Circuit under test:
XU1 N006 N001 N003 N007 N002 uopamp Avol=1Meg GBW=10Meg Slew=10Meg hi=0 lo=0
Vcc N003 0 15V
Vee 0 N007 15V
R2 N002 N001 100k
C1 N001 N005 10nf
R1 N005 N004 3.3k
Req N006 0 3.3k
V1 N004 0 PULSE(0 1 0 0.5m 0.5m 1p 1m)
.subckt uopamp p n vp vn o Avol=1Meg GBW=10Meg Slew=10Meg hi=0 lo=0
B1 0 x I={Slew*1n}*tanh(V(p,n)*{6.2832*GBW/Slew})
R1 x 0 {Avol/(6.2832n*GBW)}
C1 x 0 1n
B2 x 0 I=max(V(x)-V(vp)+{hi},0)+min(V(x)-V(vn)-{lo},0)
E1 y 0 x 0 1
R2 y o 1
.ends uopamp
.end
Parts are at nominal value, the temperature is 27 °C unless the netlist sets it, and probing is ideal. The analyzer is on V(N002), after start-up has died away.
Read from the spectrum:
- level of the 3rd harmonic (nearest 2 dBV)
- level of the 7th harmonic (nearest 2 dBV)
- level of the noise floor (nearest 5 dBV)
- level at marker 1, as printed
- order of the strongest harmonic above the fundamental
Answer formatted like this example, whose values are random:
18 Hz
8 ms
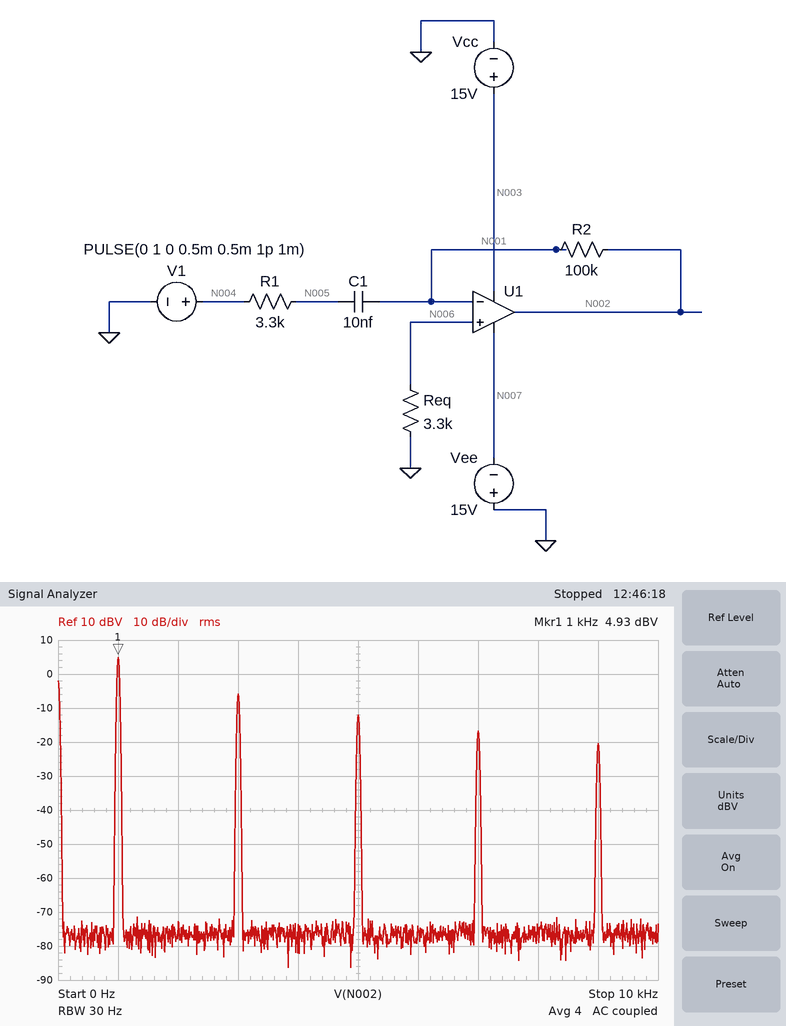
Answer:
-6 dBV
-16 dBV
-75 dBV
4.93 dBV
3
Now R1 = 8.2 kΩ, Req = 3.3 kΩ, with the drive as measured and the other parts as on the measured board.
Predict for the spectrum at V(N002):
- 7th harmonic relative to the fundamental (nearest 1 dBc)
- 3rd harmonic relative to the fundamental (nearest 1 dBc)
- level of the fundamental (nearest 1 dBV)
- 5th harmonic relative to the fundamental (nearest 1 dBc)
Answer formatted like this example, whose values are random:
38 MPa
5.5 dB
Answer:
-27 dBc
-14 dBc
4 dBV
-22 dBc
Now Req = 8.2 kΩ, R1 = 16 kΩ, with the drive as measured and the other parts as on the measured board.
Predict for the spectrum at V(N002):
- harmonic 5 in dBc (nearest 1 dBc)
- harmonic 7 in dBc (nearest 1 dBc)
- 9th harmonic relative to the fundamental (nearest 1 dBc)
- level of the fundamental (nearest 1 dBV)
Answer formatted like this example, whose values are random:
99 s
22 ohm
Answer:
-25 dBc
-31 dBc
-35 dBc
2 dBV
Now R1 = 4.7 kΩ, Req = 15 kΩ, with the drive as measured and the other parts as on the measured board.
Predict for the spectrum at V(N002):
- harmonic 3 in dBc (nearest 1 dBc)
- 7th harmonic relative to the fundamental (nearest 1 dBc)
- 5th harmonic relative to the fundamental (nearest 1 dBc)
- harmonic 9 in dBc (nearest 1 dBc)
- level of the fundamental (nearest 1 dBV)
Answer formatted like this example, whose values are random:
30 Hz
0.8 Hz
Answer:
-12 dBc
-24 dBc
-19 dBc
-28 dBc
5 dBV
